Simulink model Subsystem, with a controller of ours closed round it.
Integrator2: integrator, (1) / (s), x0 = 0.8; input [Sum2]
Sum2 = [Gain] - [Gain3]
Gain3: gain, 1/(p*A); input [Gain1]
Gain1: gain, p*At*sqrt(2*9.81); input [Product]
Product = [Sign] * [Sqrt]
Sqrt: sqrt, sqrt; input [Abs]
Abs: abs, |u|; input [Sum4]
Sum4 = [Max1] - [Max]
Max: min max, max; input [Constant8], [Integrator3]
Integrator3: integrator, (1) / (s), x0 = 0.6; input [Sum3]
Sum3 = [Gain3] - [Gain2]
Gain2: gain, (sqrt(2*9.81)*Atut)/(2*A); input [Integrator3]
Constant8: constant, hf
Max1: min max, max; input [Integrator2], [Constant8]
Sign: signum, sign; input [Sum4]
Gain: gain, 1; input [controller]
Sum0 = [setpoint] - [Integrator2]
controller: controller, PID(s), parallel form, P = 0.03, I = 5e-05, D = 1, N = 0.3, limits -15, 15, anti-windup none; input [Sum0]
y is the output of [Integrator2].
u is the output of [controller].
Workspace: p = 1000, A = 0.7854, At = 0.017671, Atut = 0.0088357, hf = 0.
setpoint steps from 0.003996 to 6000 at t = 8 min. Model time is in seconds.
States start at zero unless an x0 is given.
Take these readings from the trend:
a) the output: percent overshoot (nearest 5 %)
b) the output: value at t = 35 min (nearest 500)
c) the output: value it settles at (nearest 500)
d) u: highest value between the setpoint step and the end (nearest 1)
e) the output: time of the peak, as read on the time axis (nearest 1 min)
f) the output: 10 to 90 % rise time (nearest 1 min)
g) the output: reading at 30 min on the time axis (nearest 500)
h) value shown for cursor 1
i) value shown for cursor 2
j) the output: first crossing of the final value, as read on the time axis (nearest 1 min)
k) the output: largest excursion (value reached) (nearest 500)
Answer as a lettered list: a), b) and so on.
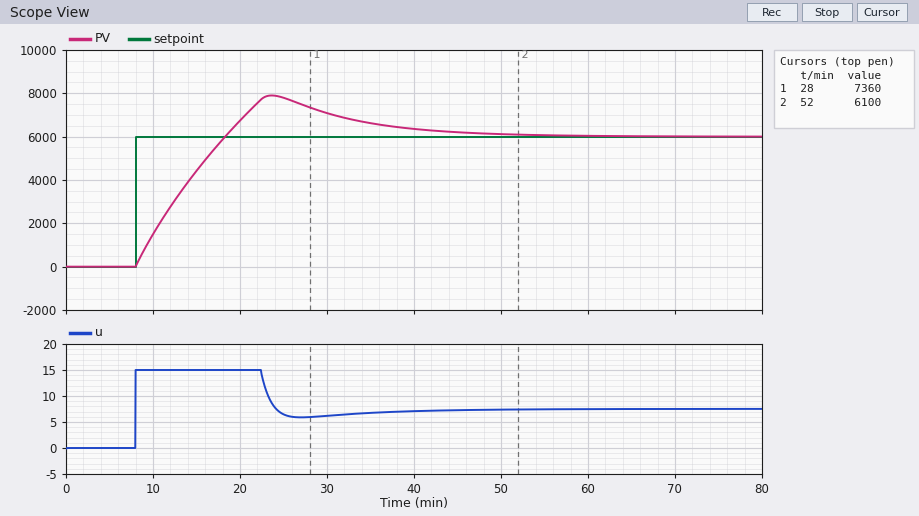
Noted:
a) 30 %
b) 6500
c) 6000
d) 15
e) 24 min
f) 8 min
g) 7000
h) 7360
i) 6100
j) 18 min
k) 8000
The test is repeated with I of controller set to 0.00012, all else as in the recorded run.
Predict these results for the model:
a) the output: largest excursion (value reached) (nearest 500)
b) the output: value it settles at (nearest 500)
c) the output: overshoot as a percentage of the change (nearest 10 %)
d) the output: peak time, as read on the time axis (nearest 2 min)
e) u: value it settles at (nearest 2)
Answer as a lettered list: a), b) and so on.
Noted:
a) 9000
b) 6000
c) 50 %
d) 26 min
e) 8
